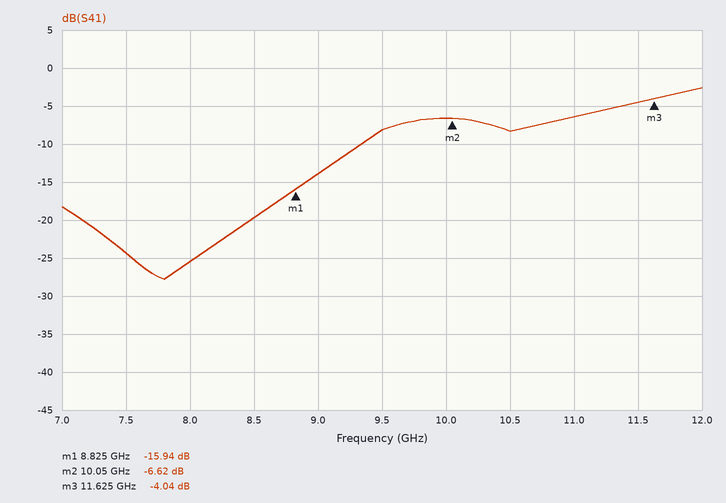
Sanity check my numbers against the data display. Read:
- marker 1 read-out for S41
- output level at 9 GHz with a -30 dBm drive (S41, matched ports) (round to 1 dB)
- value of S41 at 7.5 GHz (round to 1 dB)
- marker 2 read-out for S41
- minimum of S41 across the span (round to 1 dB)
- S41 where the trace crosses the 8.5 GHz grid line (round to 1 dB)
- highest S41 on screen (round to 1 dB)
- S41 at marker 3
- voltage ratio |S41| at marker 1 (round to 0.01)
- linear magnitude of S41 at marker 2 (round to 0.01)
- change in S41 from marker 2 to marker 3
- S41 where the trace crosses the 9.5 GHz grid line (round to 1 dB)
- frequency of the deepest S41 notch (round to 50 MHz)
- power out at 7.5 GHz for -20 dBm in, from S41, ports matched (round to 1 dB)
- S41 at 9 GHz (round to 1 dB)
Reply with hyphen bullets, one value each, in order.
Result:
- -15.94 dB
- -44 dBm
- -24 dB
- -6.62 dB
- -28 dB
- -20 dB
- -3 dB
- -4.04 dB
- 0.16
- 0.47
- 2.58 dB
- -8 dB
- 7.80 GHz
- -44 dBm
- -14 dB
